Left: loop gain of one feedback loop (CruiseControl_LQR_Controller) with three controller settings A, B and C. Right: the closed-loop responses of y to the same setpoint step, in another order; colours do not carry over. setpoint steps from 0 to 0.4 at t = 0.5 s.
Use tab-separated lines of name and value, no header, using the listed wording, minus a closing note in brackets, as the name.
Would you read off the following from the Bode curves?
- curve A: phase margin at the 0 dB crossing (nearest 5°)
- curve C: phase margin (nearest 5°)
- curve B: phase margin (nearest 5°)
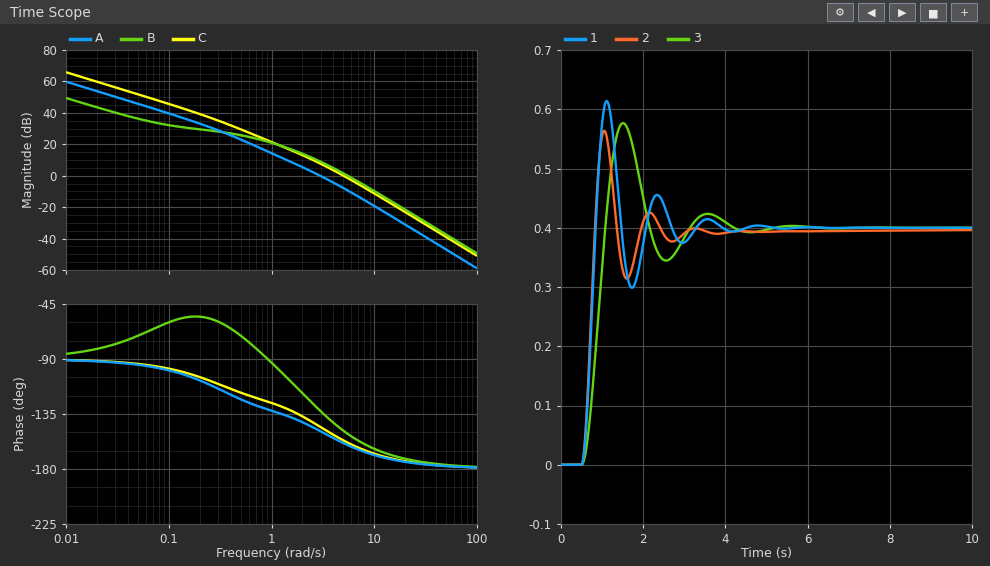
curve A: phase margin at the 0 dB crossing	30°
curve C: phase margin	25°
curve B: phase margin	30°
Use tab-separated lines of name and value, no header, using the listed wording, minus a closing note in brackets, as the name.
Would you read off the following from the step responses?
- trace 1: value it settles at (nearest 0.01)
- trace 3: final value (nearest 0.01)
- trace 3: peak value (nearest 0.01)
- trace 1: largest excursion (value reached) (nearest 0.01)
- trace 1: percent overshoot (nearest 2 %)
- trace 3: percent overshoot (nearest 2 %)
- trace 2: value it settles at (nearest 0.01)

trace 1: value it settles at	0.40
trace 3: final value	0.40
trace 3: peak value	0.58
trace 1: largest excursion (value reached)	0.61
trace 1: percent overshoot	54 %
trace 3: percent overshoot	44 %
trace 2: value it settles at	0.40
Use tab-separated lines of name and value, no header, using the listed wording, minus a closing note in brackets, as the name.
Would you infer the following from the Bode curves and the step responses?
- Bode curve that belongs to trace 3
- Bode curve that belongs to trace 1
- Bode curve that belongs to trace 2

Bode curve that belongs to trace 3	A
Bode curve that belongs to trace 1	C
Bode curve that belongs to trace 2	B
